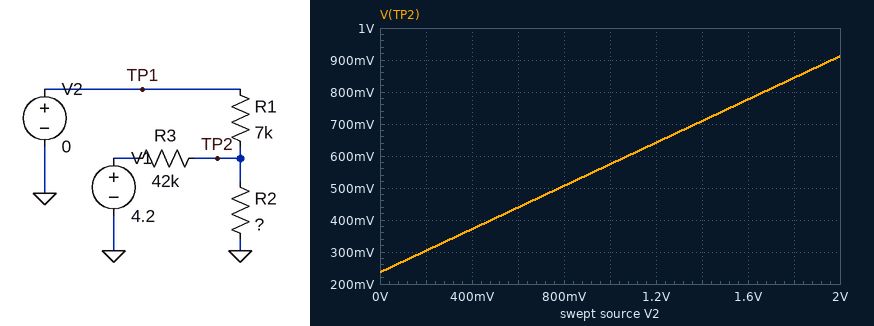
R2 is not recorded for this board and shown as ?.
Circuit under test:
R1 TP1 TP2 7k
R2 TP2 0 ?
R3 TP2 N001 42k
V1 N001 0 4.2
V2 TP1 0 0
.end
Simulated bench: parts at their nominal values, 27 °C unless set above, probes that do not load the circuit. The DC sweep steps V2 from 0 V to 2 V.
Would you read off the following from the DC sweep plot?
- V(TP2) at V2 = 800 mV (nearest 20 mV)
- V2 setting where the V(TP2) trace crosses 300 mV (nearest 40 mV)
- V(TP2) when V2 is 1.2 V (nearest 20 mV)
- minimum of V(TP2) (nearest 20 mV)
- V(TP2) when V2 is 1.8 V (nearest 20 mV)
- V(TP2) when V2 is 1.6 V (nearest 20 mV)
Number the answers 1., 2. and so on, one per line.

1. 500 mV
2. 200 mV
3. 640 mV
4. 240 mV
5. 840 mV
6. 780 mV
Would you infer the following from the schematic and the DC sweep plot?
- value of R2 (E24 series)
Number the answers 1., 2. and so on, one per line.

1. 3.9 kΩ
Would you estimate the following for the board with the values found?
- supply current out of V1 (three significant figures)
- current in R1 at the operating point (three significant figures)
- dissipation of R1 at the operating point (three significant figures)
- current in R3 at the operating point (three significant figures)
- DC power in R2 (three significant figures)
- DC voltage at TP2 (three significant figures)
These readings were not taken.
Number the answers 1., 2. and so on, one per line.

1. 94.4 µA
2. 33.8 µA
3. 7.98 µW
4. 94.4 µA
5. 14.3 µW
6. 236 mV
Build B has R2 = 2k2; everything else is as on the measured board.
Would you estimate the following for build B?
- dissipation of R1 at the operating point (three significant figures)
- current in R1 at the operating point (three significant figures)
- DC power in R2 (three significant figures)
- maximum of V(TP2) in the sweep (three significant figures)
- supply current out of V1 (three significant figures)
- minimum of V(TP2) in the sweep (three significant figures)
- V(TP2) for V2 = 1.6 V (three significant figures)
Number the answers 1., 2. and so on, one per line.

1. 3.70 µW
2. 23.0 µA
3. 11.8 µW
4. 621 mV
5. 96.2 µA
6. 161 mV
7. 529 mV
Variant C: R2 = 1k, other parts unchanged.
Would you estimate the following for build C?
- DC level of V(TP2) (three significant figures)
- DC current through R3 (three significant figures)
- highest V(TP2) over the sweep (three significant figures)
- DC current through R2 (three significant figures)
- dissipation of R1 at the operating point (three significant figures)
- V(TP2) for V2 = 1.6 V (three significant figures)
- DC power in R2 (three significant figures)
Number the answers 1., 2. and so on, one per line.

1. 85.7 mV
2. 98.0 µA
3. 331 mV
4. 85.7 µA
5. 1.05 µW
6. 282 mV
7. 7.35 µW
